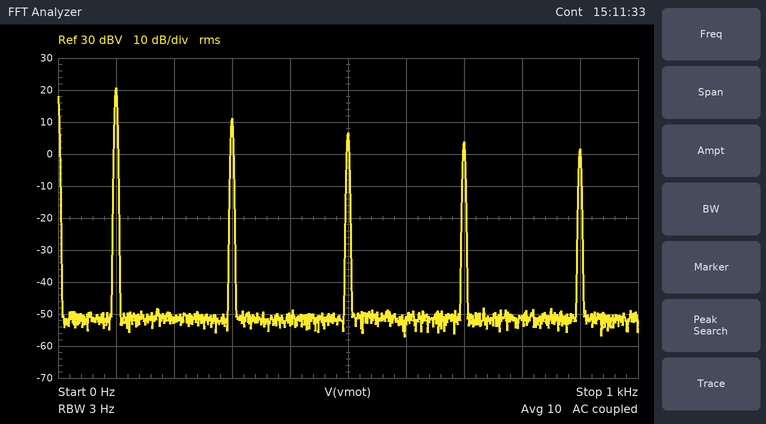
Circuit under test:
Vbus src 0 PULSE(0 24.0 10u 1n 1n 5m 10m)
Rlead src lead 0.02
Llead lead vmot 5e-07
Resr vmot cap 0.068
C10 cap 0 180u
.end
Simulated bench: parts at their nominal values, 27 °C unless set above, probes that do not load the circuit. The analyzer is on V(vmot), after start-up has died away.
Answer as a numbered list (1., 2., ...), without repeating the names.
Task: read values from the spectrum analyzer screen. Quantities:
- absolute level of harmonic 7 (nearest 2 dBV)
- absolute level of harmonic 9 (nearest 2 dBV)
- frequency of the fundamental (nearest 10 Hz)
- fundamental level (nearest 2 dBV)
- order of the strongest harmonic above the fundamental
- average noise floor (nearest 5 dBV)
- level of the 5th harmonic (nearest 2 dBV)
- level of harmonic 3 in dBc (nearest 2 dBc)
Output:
1. 4 dBV
2. 2 dBV
3. 100 Hz
4. 20 dBV
5. 3
6. -50 dBV
7. 6 dBV
8. -10 dBc
